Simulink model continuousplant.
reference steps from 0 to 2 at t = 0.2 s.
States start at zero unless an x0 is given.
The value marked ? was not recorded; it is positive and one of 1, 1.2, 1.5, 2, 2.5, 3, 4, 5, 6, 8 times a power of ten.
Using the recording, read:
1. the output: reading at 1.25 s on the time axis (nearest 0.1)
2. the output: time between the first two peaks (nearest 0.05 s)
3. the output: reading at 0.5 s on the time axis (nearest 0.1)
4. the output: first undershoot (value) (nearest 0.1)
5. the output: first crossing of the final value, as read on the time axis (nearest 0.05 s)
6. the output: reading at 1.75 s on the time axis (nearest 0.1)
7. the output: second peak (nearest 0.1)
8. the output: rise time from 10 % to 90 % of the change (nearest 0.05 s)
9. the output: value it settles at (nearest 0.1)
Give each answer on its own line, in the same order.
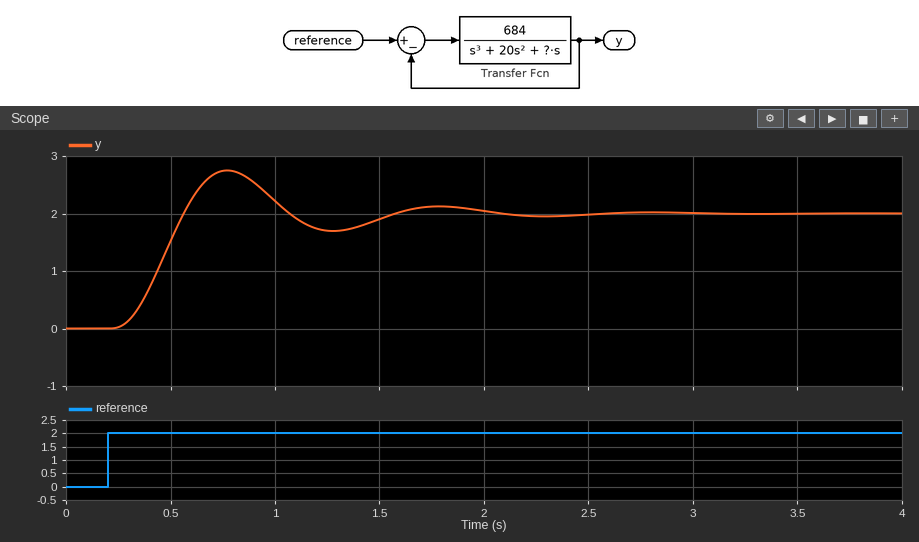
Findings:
1.7
1.00 s
1.5
1.7
0.55 s
2.1
2.1
0.20 s
2.0
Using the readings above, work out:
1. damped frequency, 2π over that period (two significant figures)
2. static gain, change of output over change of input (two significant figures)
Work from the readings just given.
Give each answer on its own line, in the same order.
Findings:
6.3 rad/s
1.0
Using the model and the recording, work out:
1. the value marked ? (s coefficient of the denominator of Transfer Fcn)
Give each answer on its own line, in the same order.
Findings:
100
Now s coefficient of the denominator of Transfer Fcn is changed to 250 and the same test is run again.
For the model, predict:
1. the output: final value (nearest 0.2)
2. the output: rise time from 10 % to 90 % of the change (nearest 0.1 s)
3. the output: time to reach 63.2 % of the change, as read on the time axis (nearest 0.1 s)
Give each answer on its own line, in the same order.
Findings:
2.0
0.6 s
0.6 s
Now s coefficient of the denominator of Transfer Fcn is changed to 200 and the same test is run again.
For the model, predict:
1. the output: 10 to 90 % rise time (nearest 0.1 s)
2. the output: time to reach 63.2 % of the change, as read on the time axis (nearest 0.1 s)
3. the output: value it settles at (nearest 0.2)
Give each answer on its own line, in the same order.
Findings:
0.4 s
0.5 s
2.0
